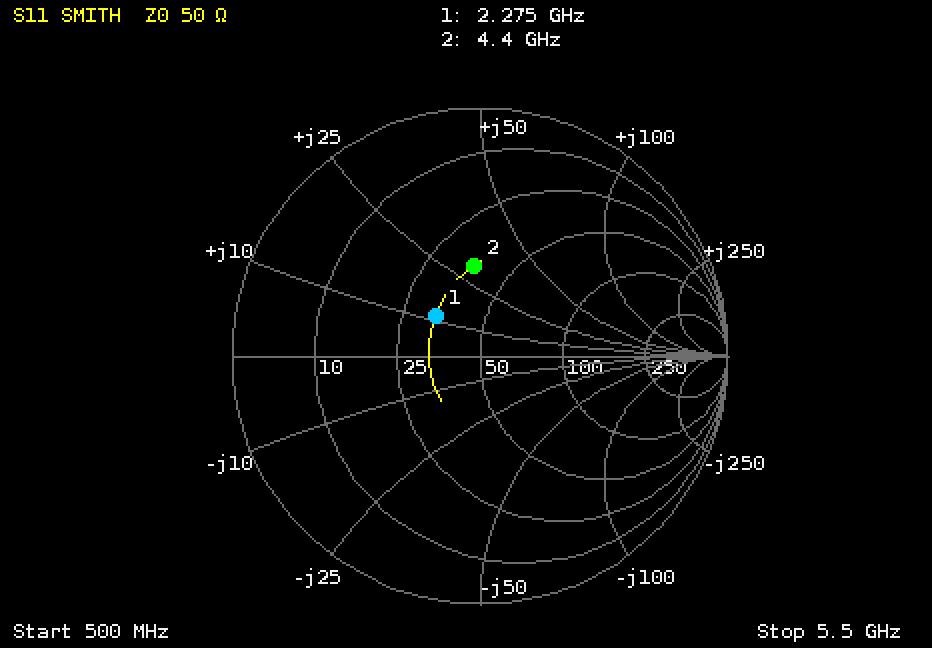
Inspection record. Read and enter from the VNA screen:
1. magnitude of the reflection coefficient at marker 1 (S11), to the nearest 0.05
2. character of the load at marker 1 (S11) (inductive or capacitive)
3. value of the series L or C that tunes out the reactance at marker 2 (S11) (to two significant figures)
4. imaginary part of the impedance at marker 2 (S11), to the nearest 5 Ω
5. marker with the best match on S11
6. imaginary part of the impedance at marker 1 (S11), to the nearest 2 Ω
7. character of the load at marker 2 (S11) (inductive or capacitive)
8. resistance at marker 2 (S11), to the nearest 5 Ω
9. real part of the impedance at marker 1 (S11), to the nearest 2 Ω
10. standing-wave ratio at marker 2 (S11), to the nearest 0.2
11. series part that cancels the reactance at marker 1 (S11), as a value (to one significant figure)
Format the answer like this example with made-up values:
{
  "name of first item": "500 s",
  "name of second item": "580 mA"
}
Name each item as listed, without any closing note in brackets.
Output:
{
  "magnitude of the reflection coefficient at marker 1 (S11), to the nearest 0.05": "0.25",
  "character of the load at marker 1 (S11)": "inductive",
  "value of the series L or C that tunes out the reactance at marker 2 (S11)": "1.2 pF",
  "imaginary part of the impedance at marker 2 (S11), to the nearest 5 Ω": "+30 Ω",
  "marker with the best match on S11": "marker 1",
  "imaginary part of the impedance at marker 1 (S11), to the nearest 2 Ω": "+12 Ω",
  "character of the load at marker 2 (S11)": "inductive",
  "resistance at marker 2 (S11), to the nearest 5 Ω": "35 Ω",
  "real part of the impedance at marker 1 (S11), to the nearest 2 Ω": "34 Ω",
  "standing-wave ratio at marker 2 (S11), to the nearest 0.2": "2.2",
  "series part that cancels the reactance at marker 1 (S11), as a value": "6 pF"
}
